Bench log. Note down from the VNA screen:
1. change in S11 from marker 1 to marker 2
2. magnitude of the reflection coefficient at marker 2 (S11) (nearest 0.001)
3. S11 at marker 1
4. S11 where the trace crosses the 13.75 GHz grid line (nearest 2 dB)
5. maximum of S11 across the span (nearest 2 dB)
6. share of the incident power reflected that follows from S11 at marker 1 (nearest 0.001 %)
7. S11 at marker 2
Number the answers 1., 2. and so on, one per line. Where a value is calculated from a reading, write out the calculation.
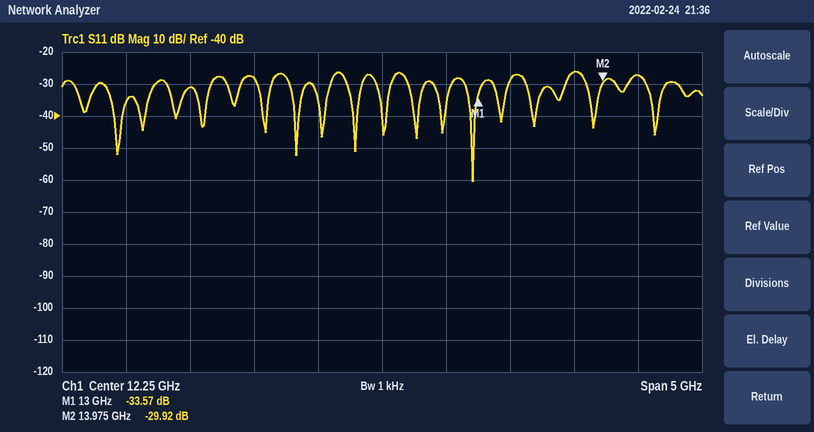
1. -29.92 − (-33.57) = 3.65 dB
2. 10^(-29.92/20) ≈ 0.032
3. -33.57 dB
4. -26 dB
5. -26 dB
6. 10^(-33.57/10) ≈ 0.044 %
7. -29.92 dB
